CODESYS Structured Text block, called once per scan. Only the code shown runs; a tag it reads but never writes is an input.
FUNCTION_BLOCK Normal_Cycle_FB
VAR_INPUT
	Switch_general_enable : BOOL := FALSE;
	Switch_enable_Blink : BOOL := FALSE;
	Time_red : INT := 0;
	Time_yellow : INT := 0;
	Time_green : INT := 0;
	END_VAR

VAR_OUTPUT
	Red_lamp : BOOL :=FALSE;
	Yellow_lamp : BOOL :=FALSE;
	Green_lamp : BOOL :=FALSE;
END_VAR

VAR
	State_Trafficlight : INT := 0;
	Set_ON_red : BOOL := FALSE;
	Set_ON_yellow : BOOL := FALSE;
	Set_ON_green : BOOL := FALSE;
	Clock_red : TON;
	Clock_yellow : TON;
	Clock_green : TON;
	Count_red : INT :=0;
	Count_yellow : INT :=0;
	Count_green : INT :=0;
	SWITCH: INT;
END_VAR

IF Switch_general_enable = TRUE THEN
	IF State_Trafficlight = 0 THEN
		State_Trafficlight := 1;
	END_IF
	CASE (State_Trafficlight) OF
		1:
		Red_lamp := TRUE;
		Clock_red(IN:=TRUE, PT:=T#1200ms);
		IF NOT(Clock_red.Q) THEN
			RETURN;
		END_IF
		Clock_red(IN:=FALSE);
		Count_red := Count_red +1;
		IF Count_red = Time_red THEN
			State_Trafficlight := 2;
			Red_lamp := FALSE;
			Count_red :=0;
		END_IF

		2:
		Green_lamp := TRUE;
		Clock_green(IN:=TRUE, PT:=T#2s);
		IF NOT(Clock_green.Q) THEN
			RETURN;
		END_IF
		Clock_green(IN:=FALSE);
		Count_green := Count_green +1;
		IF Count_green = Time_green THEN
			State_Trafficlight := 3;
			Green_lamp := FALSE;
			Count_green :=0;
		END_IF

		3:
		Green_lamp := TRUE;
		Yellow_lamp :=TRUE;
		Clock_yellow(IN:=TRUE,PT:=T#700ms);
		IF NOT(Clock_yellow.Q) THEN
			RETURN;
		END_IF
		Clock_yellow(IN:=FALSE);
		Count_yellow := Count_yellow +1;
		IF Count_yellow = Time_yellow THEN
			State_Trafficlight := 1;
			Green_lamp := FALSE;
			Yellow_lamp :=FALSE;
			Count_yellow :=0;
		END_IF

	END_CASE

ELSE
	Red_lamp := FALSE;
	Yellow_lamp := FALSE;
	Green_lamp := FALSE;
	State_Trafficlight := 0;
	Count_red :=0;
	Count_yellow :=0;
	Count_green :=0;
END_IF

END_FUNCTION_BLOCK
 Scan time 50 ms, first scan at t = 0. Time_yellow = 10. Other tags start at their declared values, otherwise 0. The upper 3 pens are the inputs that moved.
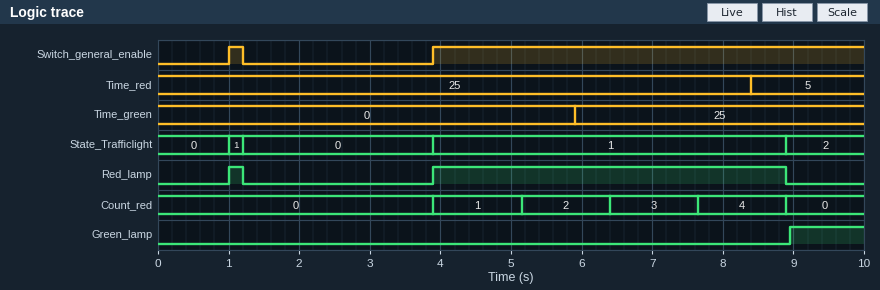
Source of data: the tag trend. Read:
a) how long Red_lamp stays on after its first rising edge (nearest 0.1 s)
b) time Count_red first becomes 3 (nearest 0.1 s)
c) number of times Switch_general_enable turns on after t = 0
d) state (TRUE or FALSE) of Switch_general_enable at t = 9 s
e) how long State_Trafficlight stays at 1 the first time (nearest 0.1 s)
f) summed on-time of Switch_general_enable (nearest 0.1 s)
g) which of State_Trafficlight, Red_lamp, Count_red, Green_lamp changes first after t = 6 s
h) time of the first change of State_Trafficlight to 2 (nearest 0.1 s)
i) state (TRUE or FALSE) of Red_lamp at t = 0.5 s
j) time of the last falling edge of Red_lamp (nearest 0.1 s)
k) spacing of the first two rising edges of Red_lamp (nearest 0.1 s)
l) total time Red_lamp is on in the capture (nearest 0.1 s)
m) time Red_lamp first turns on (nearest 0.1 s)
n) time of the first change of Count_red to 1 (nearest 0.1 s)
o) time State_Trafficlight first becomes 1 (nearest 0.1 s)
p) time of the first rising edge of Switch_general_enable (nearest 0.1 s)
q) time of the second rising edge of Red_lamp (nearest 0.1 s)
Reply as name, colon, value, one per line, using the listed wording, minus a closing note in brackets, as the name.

how long Red_lamp stays on after its first rising edge: 0.2 s
time Count_red first becomes 3: 6.4 s
number of times Switch_general_enable turns on after t = 0: 2
state (TRUE or FALSE) of Switch_general_enable at t = 9 s: TRUE
how long State_Trafficlight stays at 1 the first time: 0.2 s
summed on-time of Switch_general_enable: 6.3 s
which of State_Trafficlight, Red_lamp, Count_red, Green_lamp changes first after t = 6 s: Count_red
time of the first change of State_Trafficlight to 2: 8.9 s
state (TRUE or FALSE) of Red_lamp at t = 0.5 s: FALSE
time of the last falling edge of Red_lamp: 8.9 s
spacing of the first two rising edges of Red_lamp: 2.9 s
total time Red_lamp is on in the capture: 5.2 s
time Red_lamp first turns on: 1.0 s
time of the first change of Count_red to 1: 3.9 s
time State_Trafficlight first becomes 1: 1.0 s
time of the first rising edge of Switch_general_enable: 1.0 s
time of the second rising edge of Red_lamp: 3.9 s
